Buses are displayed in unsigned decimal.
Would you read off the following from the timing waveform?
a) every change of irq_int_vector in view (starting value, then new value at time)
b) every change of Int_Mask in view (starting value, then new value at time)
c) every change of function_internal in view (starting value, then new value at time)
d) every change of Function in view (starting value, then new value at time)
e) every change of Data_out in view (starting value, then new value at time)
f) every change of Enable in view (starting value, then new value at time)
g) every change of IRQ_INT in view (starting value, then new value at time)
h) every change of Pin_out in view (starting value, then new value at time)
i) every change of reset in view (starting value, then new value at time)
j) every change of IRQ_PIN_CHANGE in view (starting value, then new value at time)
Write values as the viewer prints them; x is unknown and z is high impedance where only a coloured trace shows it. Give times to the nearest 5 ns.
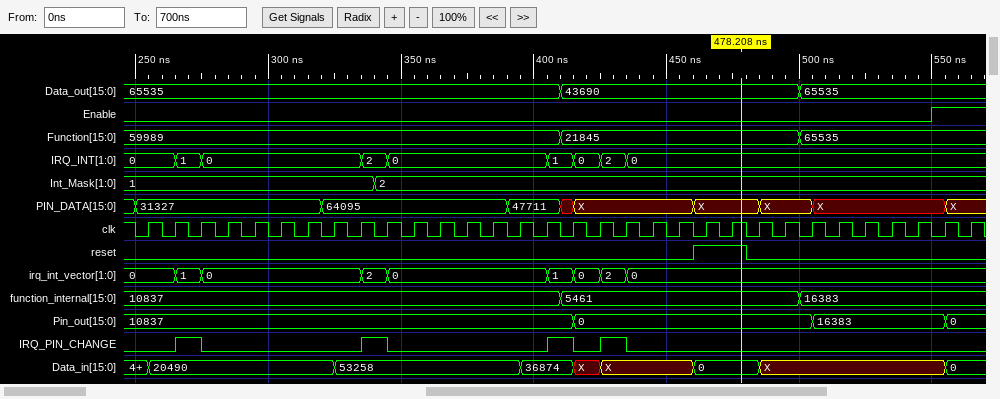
0, 1 at 265 ns, 0 at 275 ns, 2 at 335 ns, 0 at 345 ns, 1 at 405 ns, 0 at 415 ns, 2 at 425 ns, 0 at 435 ns
1, 2 at 340 ns
10837, 5461 at 410 ns, 16383 at 500 ns
59989, 21845 at 410 ns, 65535 at 500 ns
65535, 43690 at 410 ns, 65535 at 500 ns
0, 1 at 550 ns
0, 1 at 265 ns, 0 at 275 ns, 2 at 335 ns, 0 at 345 ns, 1 at 405 ns, 0 at 415 ns, 2 at 425 ns, 0 at 435 ns
10837, 0 at 415 ns, 16383 at 505 ns, 0 at 555 ns
0, 1 at 460 ns, 0 at 480 ns
0, 1 at 265 ns, 0 at 275 ns, 1 at 335 ns, 0 at 345 ns, 1 at 405 ns, 0 at 415 ns, 1 at 425 ns, 0 at 435 ns
